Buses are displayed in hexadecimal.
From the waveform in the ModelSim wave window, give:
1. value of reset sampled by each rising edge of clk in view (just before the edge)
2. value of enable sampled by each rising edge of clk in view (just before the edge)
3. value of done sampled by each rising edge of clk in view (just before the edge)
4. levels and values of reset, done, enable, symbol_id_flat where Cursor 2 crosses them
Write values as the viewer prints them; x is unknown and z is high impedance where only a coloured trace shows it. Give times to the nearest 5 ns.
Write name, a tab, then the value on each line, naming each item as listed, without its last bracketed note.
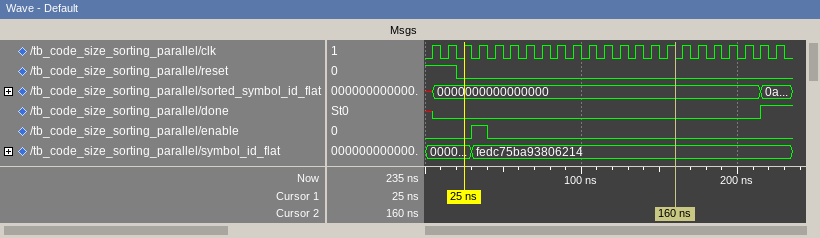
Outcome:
value of reset sampled by each rising edge of clk in view	1 1 0 0 0 0 0 0 0 0 0 0 0 0 0 0 0 0 0 0 0 0 0
value of enable sampled by each rising edge of clk in view	0 0 0 1 0 0 0 0 0 0 0 0 0 0 0 0 0 0 0 0 0 0 0
value of done sampled by each rising edge of clk in view	x 0 0 0 0 0 0 0 0 0 0 0 0 0 0 0 0 0 0 0 0 0 1
levels and values of reset, done, enable, symbol_id_flat where Cursor 2 crosses them	reset=0, done=0, enable=0, symbol_id_flat=fedc75ba93806214
